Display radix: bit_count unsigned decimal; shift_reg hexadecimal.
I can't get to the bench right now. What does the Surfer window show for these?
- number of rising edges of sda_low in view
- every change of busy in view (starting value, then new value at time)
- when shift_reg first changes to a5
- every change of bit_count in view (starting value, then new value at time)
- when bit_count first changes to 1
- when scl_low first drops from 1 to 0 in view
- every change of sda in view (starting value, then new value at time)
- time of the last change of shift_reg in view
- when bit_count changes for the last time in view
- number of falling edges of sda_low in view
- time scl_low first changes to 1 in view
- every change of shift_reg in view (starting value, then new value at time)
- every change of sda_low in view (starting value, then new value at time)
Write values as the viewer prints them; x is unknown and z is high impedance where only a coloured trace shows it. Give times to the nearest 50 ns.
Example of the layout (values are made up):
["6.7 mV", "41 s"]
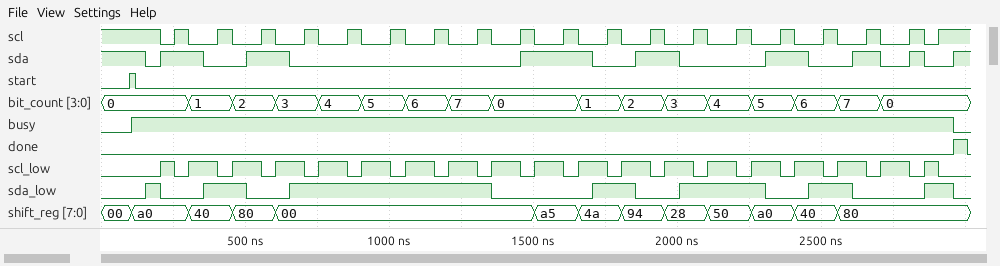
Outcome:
["7", "0, 1 at 100 ns, 0 at 2950 ns", "1500 ns", "0, 1 at 300 ns, 2 at 450 ns, 3 at 600 ns, 4 at 750 ns, 5 at 900 ns, 6 at 1050 ns, 7 at 1200 ns, 0 at 1350 ns, 1 at 1650 ns, 2 at 1800 ns, 3 at 1950 ns, 4 at 2100 ns, 5 at 2250 ns, 6 at 2400 ns, 7 at 2550 ns, 0 at 2700 ns", "300 ns", "250 ns", "1, 0 at 150 ns, 1 at 200 ns, 0 at 350 ns, 1 at 500 ns, 0 at 650 ns, 1 at 1450 ns, 0 at 1700 ns, 1 at 1850 ns, 0 at 2000 ns, 1 at 2300 ns, 0 at 2450 ns, 1 at 2600 ns, 0 at 2700 ns, 1 at 2800 ns, 0 at 2850 ns, 1 at 2950 ns", "2550 ns", "2700 ns", "7", "200 ns", "00, a0 at 100 ns, 40 at 300 ns, 80 at 450 ns, 00 at 600 ns, a5 at 1500 ns, 4a at 1650 ns, 94 at 1800 ns, 28 at 1950 ns, 50 at 2100 ns, a0 at 2250 ns, 40 at 2400 ns, 80 at 2550 ns", "0, 1 at 150 ns, 0 at 200 ns, 1 at 350 ns, 0 at 500 ns, 1 at 650 ns, 0 at 1350 ns, 1 at 1700 ns, 0 at 1850 ns, 1 at 2000 ns, 0 at 2300 ns, 1 at 2450 ns, 0 at 2600 ns, 1 at 2850 ns, 0 at 2950 ns"]
